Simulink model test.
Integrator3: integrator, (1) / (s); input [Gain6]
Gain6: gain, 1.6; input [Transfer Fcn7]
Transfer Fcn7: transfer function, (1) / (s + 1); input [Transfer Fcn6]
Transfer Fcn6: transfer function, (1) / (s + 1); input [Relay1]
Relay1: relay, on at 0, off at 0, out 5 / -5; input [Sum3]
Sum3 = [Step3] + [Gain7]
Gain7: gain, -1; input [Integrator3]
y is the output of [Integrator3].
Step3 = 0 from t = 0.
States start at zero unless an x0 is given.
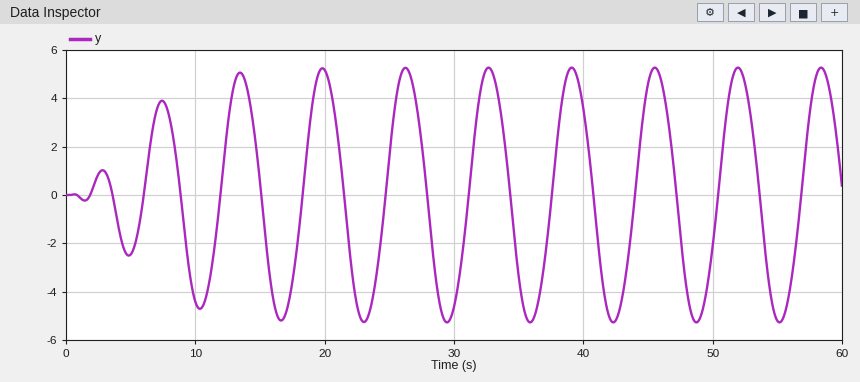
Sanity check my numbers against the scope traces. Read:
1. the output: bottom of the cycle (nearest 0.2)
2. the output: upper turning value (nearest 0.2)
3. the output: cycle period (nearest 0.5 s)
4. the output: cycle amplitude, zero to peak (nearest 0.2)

-5.2
5.2
6.5 s
5.2
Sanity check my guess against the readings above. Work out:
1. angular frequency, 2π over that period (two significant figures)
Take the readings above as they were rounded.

0.97 rad/s
